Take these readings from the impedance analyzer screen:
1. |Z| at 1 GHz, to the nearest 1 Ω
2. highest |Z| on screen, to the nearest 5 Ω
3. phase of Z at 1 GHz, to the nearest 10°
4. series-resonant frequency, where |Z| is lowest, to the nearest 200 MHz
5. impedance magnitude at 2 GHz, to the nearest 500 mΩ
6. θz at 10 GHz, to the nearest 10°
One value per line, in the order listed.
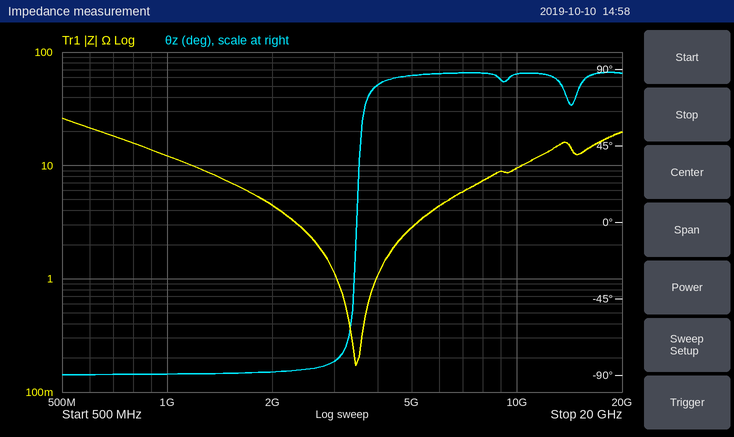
12 Ω
25 Ω
-90°
3.4 GHz
4.5 Ω
90°
